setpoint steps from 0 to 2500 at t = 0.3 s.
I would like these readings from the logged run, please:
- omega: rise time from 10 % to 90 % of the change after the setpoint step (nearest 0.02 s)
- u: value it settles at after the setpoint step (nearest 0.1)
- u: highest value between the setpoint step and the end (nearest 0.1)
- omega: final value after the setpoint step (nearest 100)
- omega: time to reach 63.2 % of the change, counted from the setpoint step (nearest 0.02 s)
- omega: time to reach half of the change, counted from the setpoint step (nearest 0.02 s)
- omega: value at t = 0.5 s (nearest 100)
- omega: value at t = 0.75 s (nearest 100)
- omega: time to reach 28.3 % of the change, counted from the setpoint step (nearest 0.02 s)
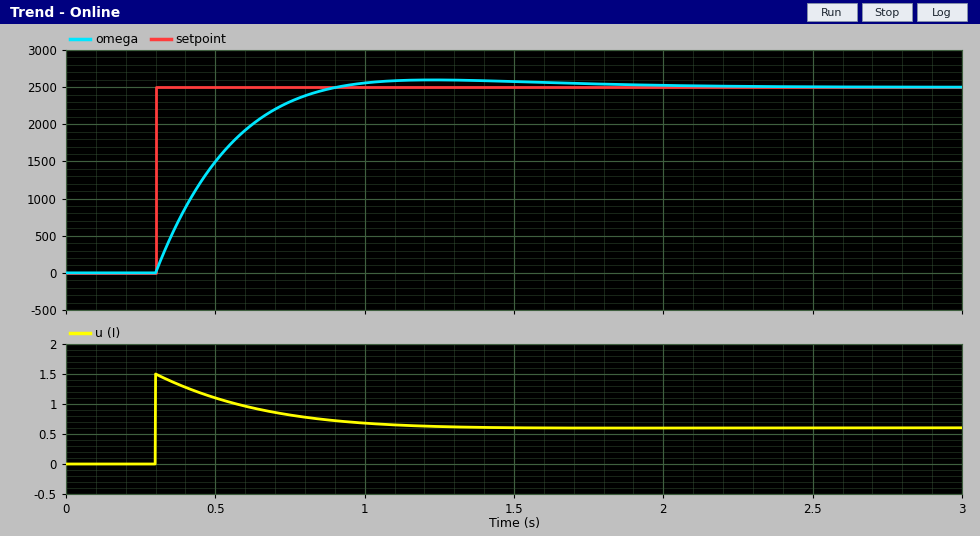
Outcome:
0.40 s
0.6
1.5
2500
0.22 s
0.16 s
1500
2300
0.08 s
